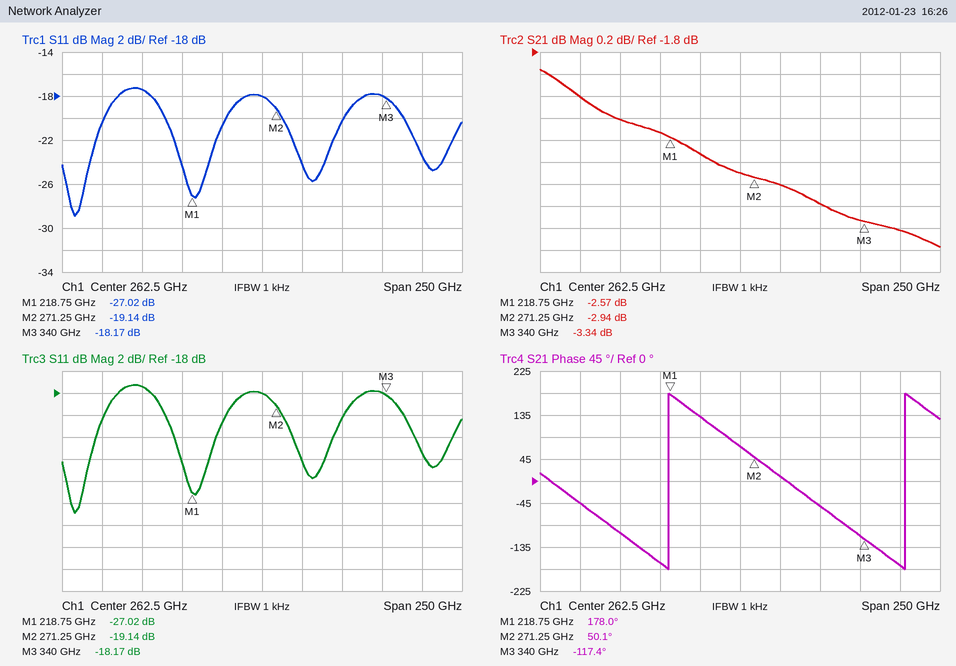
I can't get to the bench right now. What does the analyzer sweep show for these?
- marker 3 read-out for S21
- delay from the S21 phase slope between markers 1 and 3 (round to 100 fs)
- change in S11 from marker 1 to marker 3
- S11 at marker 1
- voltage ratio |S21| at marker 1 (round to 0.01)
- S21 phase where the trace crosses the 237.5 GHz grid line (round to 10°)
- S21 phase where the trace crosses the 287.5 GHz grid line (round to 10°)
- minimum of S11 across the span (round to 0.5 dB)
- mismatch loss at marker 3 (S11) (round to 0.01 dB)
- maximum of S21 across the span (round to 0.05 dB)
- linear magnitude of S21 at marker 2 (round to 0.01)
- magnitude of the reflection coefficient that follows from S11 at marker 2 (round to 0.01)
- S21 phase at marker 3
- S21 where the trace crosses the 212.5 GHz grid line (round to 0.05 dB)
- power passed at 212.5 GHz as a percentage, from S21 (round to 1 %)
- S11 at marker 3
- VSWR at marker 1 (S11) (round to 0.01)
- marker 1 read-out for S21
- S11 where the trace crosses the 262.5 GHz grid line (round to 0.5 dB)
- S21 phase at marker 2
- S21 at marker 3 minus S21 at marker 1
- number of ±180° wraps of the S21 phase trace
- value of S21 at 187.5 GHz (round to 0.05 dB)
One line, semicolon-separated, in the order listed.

-3.34 dB; 6.8 ps; 8.85 dB; -27.02 dB; 0.74; 130°; 10°; -29.0 dB; 0.07 dB; -1.95 dB; 0.71; 0.11; -117.4°; -2.55 dB; 56 %; -18.17 dB; 1.09; -2.57 dB; -18.0 dB; 50.1°; -0.77 dB; 2; -2.40 dB
